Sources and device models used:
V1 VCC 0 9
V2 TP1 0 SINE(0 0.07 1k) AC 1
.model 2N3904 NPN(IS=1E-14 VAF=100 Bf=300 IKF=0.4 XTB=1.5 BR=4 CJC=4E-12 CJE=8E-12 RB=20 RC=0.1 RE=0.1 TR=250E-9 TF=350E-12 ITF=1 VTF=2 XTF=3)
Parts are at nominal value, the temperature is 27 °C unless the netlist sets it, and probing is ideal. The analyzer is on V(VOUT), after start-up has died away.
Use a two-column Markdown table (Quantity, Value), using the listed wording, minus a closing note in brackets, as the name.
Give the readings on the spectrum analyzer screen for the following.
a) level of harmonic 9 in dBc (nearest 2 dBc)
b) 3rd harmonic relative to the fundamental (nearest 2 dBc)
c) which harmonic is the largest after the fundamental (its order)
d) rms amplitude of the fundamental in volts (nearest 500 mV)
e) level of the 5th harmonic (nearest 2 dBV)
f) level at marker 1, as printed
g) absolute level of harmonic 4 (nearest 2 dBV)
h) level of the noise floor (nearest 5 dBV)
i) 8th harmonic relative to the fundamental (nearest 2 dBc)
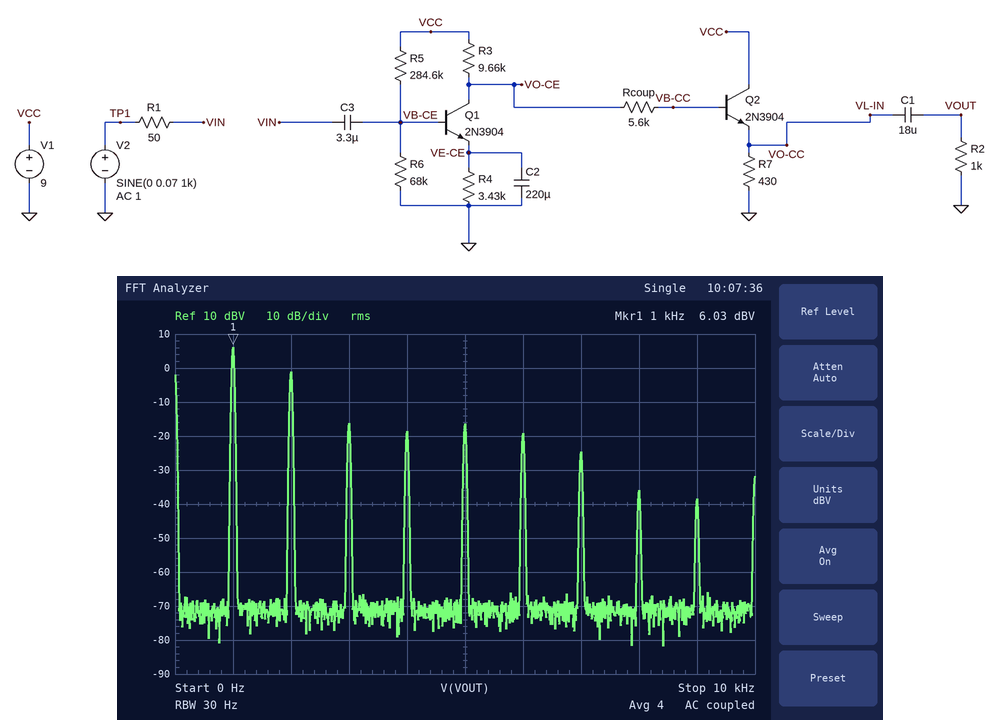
| Quantity | Value |
|---|---|
| level of harmonic 9 in dBc | -44 dBc |
| 3rd harmonic relative to the fundamental | -22 dBc |
| which harmonic is the largest after the fundamental | 2 |
| rms amplitude of the fundamental in volts | 2.0 V |
| level of the 5th harmonic | -16 dBV |
| level at marker 1, as printed | 6.03 dBV |
| absolute level of harmonic 4 | -18 dBV |
| level of the noise floor | -70 dBV |
| 8th harmonic relative to the fundamental | -42 dBc |
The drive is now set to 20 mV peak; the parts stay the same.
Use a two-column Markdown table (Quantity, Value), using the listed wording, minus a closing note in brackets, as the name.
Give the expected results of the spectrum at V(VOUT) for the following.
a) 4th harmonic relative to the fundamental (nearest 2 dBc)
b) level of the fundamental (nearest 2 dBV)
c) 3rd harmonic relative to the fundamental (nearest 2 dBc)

| Quantity | Value |
|---|---|
| 4th harmonic relative to the fundamental | -58 dBc |
| level of the fundamental | 2 dBV |
| 3rd harmonic relative to the fundamental | -34 dBc |
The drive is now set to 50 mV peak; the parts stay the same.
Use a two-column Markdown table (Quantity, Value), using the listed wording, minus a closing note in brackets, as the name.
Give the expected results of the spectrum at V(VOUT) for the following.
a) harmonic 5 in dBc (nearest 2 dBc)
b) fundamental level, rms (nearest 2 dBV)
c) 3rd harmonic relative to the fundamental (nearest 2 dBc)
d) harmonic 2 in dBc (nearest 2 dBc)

| Quantity | Value |
|---|---|
| harmonic 5 in dBc | -26 dBc |
| fundamental level, rms | 6 dBV |
| 3rd harmonic relative to the fundamental | -30 dBc |
| harmonic 2 in dBc | -10 dBc |
